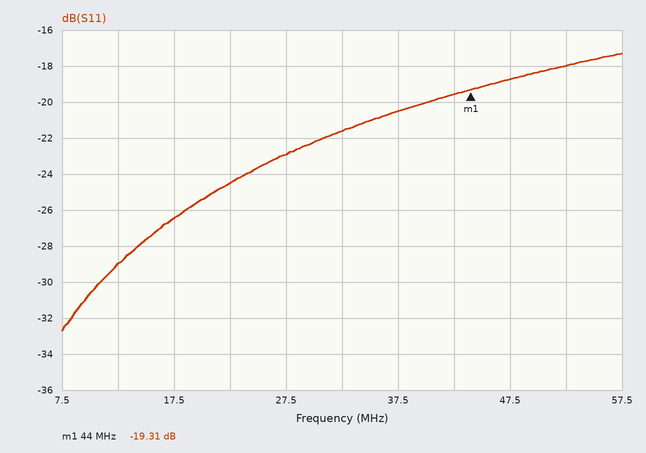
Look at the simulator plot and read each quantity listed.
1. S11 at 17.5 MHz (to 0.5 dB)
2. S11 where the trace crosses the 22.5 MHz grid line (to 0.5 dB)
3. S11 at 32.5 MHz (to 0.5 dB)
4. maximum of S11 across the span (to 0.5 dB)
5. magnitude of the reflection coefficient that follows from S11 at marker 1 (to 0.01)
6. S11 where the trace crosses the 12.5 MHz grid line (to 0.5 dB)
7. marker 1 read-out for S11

-26.5 dB
-24.5 dB
-21.5 dB
-17.5 dB
0.11
-29.0 dB
-19.31 dB
